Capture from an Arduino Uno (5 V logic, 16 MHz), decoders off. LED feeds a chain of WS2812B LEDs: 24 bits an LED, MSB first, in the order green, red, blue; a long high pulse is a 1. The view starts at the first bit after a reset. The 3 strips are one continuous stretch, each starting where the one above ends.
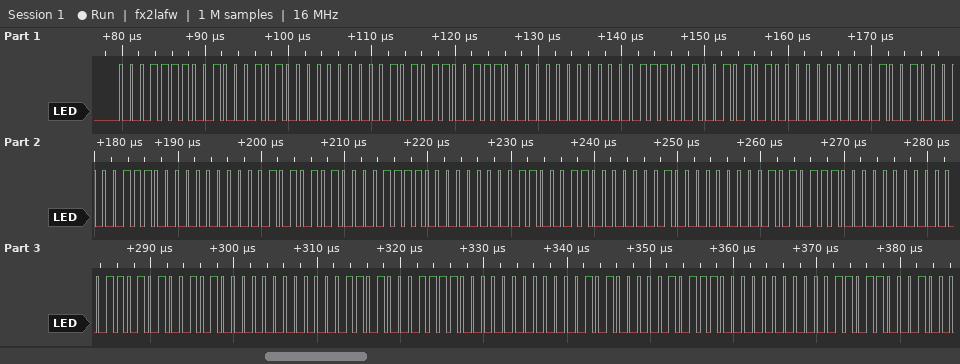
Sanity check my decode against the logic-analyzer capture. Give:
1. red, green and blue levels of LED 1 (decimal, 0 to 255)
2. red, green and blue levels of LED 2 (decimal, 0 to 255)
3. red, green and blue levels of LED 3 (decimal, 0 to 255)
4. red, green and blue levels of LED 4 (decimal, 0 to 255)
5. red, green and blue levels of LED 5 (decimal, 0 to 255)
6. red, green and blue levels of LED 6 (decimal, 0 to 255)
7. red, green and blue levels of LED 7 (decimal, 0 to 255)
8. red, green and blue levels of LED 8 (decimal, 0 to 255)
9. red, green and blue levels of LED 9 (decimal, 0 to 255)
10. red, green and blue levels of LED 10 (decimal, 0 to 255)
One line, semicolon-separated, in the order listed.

69, 30, 0; 56, 43, 0; 42, 57, 0; 28, 72, 0; 15, 85, 0; 1, 99, 0; 0, 87, 13; 0, 74, 26; 0, 60, 40; 0, 46, 54
